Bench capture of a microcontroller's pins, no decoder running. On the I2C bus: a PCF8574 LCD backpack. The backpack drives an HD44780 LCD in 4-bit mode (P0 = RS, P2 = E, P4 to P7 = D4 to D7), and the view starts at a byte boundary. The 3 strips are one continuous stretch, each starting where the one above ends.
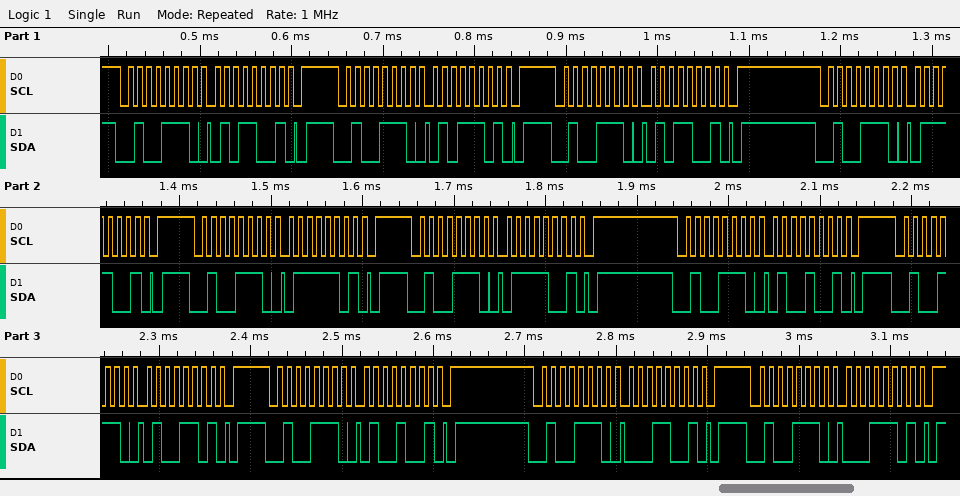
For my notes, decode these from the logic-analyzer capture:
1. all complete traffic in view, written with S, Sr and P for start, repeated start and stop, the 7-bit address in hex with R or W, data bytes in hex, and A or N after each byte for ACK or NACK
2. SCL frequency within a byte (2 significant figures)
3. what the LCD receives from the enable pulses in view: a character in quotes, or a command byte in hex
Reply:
S 27W A 59 A P S 27W A 5D A P S 27W A 59 A P S 27W A 79 A P S 27W A 7D A P S 27W A 79 A P S 27W A 49 A P S 27W A 4D A P S 27W A 49 A P S 27W A 19 A P S 27W A 1D A P
100 kHz
'W'
